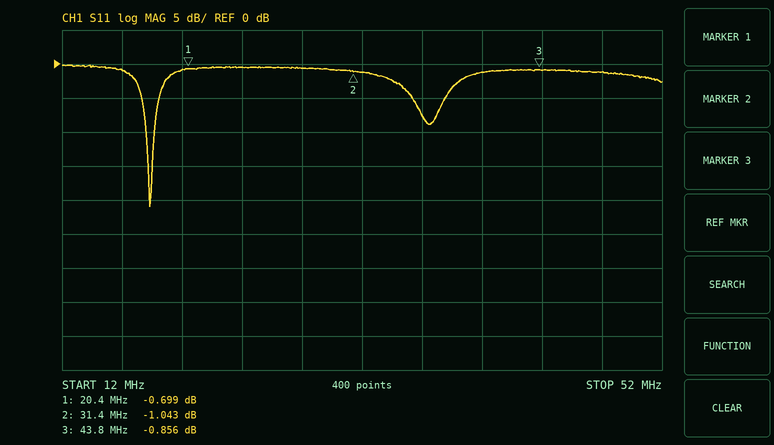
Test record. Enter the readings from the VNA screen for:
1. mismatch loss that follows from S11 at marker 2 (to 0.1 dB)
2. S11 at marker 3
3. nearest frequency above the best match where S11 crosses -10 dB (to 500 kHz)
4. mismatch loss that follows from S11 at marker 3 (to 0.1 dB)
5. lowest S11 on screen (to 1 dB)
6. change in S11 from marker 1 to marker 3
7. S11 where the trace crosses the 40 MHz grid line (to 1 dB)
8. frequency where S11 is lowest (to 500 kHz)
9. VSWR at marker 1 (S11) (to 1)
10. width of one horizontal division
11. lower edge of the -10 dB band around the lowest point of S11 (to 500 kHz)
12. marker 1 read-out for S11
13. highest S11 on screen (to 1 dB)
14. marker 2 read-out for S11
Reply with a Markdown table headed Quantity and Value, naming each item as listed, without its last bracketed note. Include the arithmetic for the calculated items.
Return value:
| Quantity | Value |
|---|---|
| mismatch loss that follows from S11 at marker 2 | −10 log10(1 − 10^(-1.043/10)) ≈ 6.7 dB |
| S11 at marker 3 | -0.856 dB |
| nearest frequency above the best match where S11 crosses -10 dB | 18.0 MHz |
| mismatch loss that follows from S11 at marker 3 | −10 log10(1 − 10^(-0.856/10)) ≈ 7.5 dB |
| lowest S11 on screen | -21 dB |
| change in S11 from marker 1 to marker 3 | -0.856 − (-0.699) = -0.157 dB |
| S11 where the trace crosses the 40 MHz grid line | -1 dB |
| frequency where S11 is lowest | 18.0 MHz |
| VSWR at marker 1 (S11) | (1 + 0.9227)/(1 − 0.9227) ≈ 25 |
| width of one horizontal division | 4 MHz |
| lower edge of the -10 dB band around the lowest point of S11 | 17.5 MHz |
| marker 1 read-out for S11 | -0.699 dB |
| highest S11 on screen | 0 dB |
| marker 2 read-out for S11 | -1.043 dB |
